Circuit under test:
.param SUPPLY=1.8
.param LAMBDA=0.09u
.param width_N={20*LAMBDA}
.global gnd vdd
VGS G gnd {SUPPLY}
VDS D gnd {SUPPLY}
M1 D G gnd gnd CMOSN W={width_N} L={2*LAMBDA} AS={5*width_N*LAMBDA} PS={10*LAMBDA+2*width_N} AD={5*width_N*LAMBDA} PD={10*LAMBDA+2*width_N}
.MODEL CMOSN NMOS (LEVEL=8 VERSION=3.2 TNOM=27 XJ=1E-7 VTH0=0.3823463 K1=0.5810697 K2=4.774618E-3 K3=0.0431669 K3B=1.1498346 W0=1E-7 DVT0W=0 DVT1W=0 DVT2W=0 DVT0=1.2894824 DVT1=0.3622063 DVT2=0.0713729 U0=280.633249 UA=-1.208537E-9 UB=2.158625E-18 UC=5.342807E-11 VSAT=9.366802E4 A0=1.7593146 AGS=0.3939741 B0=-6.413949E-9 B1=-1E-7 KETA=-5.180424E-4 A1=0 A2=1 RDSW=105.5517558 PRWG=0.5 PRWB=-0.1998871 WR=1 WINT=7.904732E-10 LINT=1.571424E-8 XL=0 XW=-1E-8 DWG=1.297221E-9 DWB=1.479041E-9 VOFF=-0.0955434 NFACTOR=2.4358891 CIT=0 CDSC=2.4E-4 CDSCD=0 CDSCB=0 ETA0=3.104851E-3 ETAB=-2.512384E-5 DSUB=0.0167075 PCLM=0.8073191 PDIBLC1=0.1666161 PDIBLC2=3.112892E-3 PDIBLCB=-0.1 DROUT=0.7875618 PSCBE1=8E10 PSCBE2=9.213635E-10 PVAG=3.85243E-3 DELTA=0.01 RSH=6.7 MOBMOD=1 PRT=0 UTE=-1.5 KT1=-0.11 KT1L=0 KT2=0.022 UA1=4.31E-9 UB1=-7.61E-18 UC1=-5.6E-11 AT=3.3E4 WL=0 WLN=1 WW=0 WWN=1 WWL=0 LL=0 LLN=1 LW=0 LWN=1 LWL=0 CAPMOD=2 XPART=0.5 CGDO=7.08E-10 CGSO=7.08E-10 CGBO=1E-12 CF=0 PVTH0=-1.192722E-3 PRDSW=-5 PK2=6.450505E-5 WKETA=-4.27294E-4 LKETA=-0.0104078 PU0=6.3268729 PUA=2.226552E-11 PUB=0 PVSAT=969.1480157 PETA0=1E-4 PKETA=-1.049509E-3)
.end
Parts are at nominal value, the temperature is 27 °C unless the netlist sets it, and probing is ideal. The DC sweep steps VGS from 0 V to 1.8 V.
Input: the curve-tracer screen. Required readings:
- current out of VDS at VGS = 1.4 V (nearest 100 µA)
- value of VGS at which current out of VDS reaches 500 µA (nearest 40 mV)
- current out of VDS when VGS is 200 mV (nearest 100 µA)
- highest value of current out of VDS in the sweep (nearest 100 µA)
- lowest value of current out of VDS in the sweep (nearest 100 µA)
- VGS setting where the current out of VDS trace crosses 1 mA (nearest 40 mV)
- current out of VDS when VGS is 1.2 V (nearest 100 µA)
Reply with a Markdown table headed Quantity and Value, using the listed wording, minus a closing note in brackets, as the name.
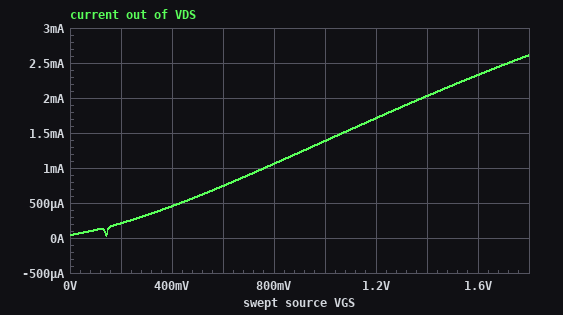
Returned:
| Quantity | Value |
|---|---|
| current out of VDS at VGS = 1.4 V | 2.0 mA |
| value of VGS at which current out of VDS reaches 500 µA | 440 mV |
| current out of VDS when VGS is 200 mV | 200 µA |
| highest value of current out of VDS in the sweep | 2.6 mA |
| lowest value of current out of VDS in the sweep | 0 A |
| VGS setting where the current out of VDS trace crosses 1 mA | 760 mV |
| current out of VDS when VGS is 1.2 V | 1.7 mA |
